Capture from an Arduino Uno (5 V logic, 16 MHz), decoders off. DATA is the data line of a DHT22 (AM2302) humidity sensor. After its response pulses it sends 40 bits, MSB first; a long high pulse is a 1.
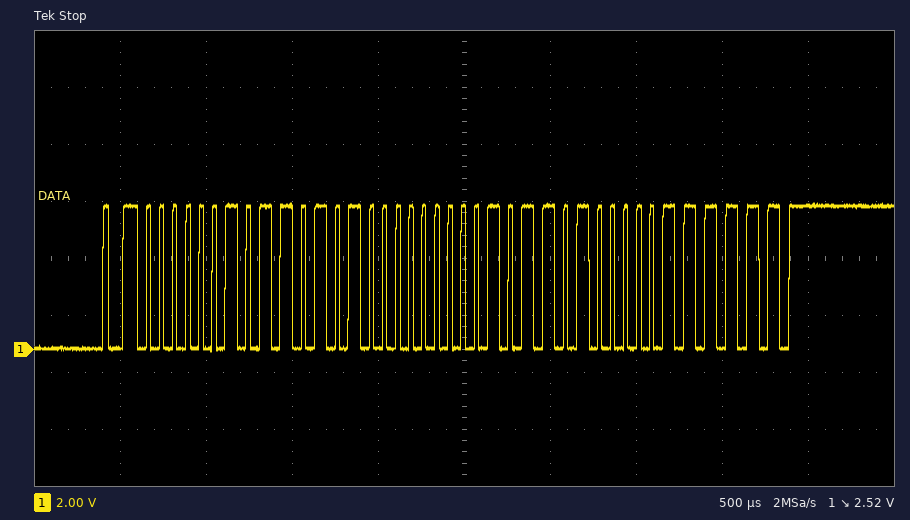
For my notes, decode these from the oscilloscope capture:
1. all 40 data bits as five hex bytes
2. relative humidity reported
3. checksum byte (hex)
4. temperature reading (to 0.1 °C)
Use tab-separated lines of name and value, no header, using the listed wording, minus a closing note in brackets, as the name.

all 40 data bits as five hex bytes	02 D4 01 68 3F
relative humidity reported	72.4 %
checksum byte	0x3F
temperature reading	36.0 °C
